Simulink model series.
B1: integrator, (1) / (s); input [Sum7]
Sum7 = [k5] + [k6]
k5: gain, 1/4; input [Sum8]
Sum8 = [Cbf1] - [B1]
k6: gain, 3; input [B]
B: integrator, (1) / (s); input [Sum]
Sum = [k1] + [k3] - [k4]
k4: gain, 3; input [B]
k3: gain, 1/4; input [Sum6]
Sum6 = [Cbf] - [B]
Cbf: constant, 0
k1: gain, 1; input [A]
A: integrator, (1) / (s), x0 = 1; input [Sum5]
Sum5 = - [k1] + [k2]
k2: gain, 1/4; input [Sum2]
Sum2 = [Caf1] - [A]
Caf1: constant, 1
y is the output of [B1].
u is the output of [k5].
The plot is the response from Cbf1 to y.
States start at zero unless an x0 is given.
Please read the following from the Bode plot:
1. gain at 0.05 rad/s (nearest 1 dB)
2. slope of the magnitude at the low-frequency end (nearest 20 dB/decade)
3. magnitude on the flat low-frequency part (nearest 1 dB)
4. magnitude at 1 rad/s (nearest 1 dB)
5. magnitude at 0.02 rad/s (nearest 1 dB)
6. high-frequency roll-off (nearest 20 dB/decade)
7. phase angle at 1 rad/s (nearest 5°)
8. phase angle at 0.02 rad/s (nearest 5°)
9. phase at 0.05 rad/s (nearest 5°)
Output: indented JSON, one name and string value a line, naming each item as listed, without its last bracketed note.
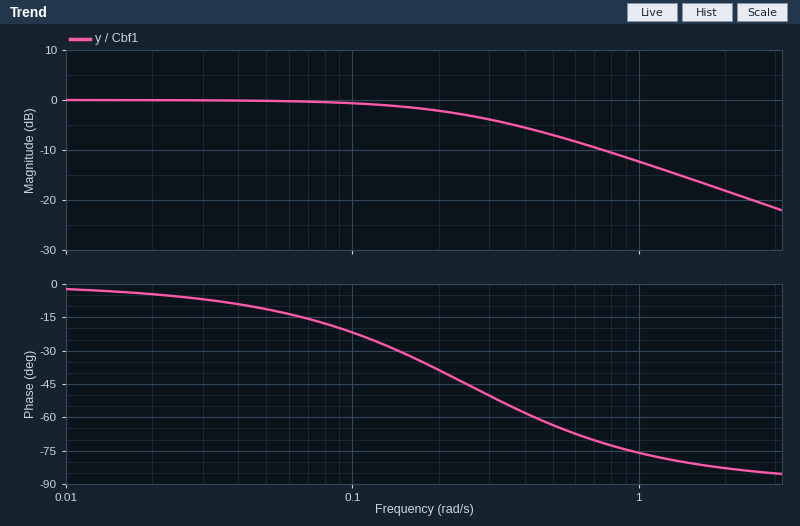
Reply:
{
  "gain at 0.05 rad/s": "0 dB",
  "slope of the magnitude at the low-frequency end": "0 dB/decade",
  "magnitude on the flat low-frequency part": "0 dB",
  "magnitude at 1 rad/s": "-12 dB",
  "magnitude at 0.02 rad/s": "0 dB",
  "high-frequency roll-off": "-20 dB/decade",
  "phase angle at 1 rad/s": "-75°",
  "phase angle at 0.02 rad/s": "-5°",
  "phase at 0.05 rad/s": "-10°"
}
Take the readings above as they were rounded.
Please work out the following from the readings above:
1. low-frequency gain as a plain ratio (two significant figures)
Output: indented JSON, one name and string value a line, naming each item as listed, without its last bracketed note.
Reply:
{
  "low-frequency gain as a plain ratio": "1.0"
}
